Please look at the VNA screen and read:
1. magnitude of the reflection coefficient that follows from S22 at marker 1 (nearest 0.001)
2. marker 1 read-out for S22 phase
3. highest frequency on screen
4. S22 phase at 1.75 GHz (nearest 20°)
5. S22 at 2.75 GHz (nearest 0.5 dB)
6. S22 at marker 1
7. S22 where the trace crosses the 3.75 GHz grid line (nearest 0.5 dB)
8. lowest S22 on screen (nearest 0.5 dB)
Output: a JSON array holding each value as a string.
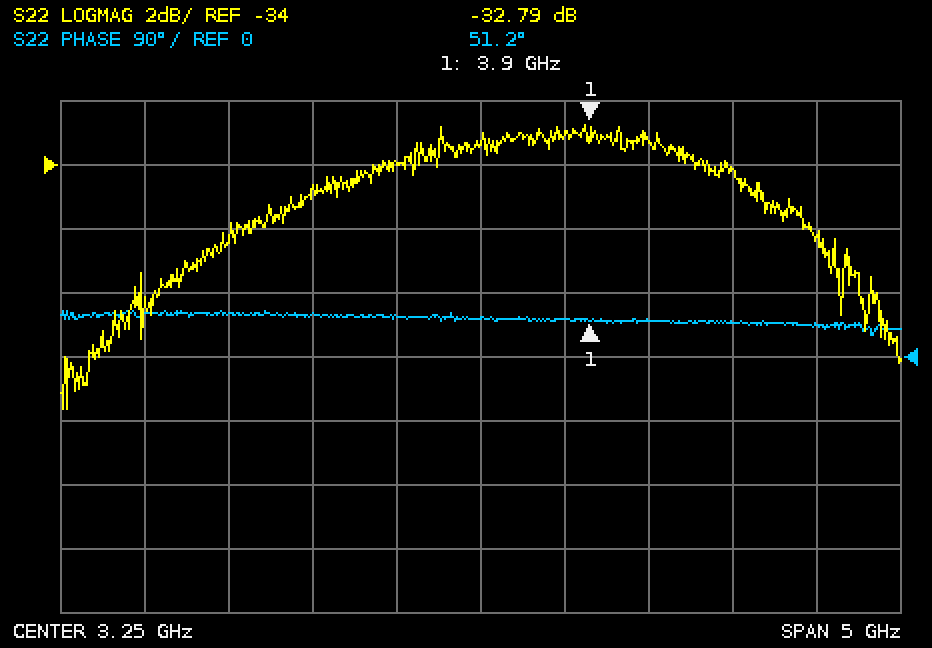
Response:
["0.023", "51.2°", "5.75 GHz", "60°", "-34.0 dB", "-32.79 dB", "-33.0 dB", "-41.5 dB"]
